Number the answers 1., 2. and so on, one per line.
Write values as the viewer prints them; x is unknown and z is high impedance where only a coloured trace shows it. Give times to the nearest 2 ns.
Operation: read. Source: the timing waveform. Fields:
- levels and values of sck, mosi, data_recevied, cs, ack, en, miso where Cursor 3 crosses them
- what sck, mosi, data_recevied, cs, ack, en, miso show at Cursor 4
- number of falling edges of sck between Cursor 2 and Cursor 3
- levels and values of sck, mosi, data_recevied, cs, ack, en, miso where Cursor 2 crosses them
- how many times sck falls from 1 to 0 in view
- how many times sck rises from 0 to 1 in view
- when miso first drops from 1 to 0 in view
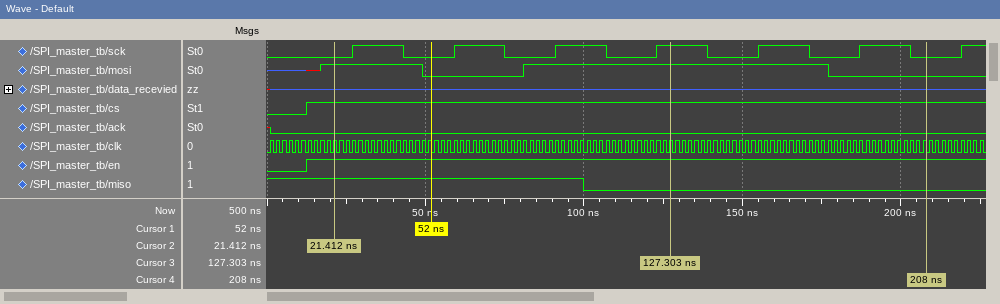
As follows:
1. sck=1, mosi=1, data_recevied=z, cs=1, ack=0, en=1, miso=0
2. sck=0, mosi=0, data_recevied=z, cs=1, ack=0, en=1, miso=0
3. 3
4. sck=0, mosi=1, data_recevied=z, cs=1, ack=0, en=1, miso=1
5. 6
6. 7
7. 100 ns
